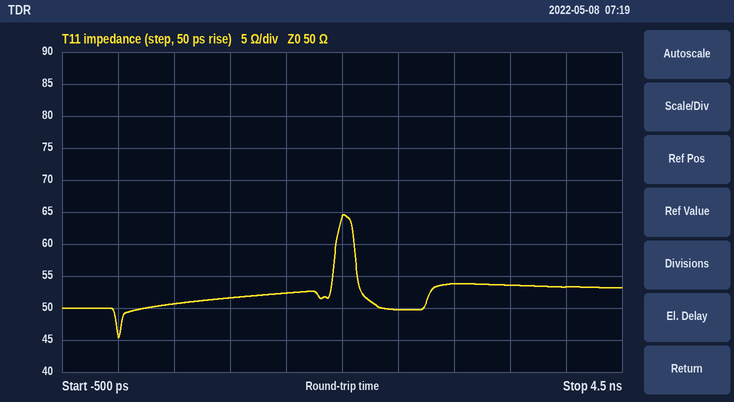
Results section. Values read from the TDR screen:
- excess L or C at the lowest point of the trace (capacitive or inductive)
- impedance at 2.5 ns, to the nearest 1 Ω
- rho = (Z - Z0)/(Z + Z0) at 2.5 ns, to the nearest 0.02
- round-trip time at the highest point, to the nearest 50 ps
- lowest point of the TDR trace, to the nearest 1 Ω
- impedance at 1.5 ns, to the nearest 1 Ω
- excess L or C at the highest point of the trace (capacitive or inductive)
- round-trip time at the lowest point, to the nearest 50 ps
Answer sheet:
capacitive
50 Ω
0.00
2.00 ns
45 Ω
52 Ω
inductive
0 ps
